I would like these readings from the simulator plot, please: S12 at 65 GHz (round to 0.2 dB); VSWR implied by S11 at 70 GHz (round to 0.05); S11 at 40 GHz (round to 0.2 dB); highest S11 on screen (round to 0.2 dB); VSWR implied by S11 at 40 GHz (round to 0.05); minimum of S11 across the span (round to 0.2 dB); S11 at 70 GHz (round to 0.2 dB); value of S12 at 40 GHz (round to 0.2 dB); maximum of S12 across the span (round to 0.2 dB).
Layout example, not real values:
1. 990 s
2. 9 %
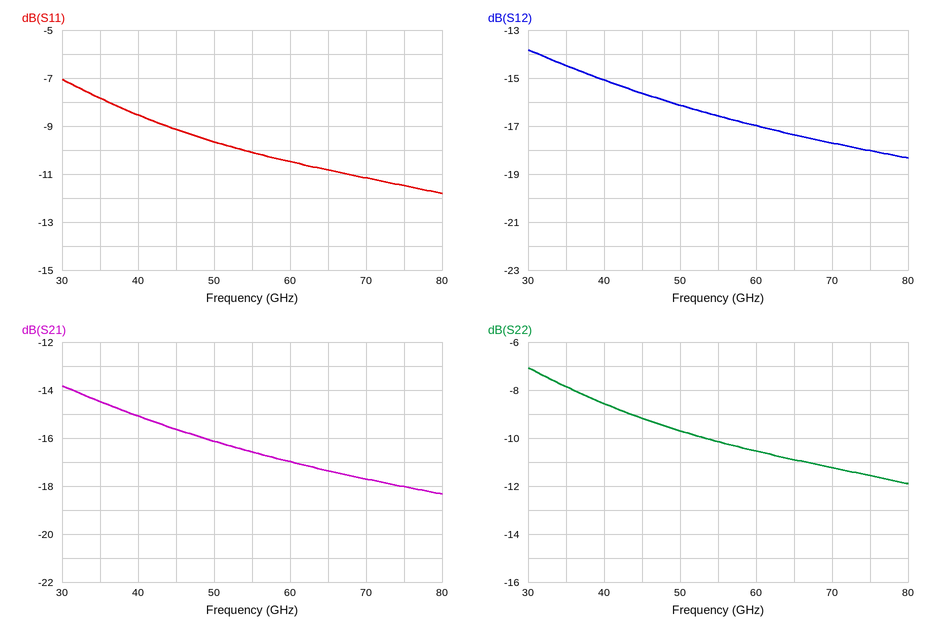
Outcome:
1. -17.4 dB
2. 1.75
3. -8.6 dB
4. -7.0 dB
5. 2.20
6. -11.8 dB
7. -11.2 dB
8. -15.0 dB
9. -13.8 dB
